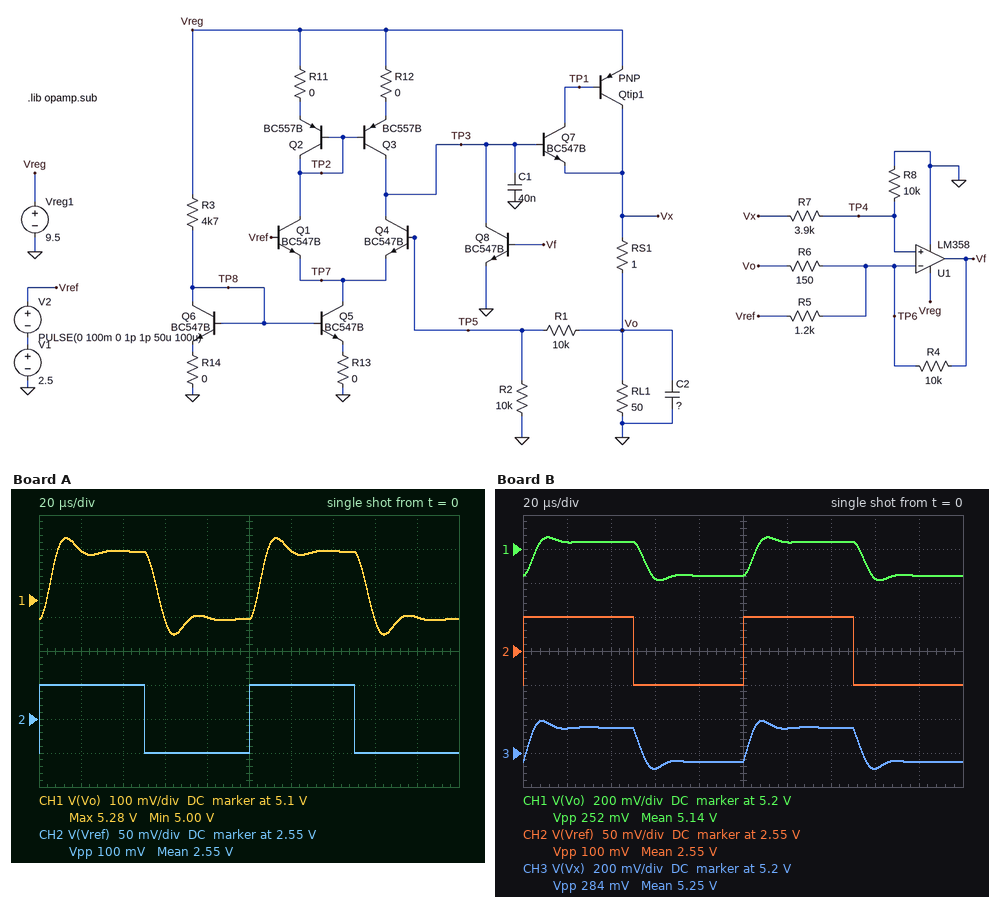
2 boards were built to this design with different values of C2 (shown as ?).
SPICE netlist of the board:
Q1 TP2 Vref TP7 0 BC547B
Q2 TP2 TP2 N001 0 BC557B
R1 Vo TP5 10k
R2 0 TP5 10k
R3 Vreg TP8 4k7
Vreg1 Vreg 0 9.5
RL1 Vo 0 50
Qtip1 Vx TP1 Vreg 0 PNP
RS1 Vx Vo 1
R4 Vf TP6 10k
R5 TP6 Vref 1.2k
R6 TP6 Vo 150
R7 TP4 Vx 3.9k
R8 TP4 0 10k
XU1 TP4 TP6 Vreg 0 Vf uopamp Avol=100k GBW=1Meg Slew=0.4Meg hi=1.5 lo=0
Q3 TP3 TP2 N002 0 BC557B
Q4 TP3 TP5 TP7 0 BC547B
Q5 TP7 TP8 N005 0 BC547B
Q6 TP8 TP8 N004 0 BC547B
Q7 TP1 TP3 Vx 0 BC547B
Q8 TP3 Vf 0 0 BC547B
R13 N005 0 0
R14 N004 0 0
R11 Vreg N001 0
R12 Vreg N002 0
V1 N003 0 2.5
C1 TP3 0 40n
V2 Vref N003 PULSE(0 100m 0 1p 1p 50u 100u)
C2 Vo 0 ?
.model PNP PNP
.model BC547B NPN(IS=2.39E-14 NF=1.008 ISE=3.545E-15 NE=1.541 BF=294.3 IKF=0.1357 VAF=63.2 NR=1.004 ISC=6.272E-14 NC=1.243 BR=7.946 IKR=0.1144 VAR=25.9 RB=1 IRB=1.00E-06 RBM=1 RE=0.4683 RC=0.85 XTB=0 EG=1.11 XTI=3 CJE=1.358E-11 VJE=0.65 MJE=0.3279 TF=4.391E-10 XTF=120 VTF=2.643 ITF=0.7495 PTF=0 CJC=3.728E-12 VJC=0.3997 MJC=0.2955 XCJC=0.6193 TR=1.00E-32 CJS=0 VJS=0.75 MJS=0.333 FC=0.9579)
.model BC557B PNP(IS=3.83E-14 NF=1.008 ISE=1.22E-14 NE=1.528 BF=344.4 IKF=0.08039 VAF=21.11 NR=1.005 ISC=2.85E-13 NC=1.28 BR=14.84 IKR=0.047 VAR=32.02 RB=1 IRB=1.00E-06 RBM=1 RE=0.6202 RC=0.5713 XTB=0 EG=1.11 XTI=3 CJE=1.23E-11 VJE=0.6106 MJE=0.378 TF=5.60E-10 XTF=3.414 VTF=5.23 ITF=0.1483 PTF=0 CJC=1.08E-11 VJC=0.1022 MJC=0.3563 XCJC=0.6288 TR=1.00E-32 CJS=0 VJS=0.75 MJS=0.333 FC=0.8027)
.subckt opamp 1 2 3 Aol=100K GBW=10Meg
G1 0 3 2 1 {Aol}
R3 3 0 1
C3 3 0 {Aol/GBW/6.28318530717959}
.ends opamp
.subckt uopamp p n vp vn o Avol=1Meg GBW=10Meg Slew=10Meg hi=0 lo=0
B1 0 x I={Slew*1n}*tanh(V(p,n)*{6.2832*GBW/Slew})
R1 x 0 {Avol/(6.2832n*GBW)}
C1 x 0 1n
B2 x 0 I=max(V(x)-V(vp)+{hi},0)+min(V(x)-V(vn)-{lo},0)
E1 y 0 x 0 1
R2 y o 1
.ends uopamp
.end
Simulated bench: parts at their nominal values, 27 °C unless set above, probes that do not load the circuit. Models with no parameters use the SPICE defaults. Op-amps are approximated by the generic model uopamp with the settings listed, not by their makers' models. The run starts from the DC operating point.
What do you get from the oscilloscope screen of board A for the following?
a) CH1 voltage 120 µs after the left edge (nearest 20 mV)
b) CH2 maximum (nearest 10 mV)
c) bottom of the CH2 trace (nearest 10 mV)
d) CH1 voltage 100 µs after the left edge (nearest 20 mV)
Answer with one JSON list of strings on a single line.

["5.24 V", "2.60 V", "2.50 V", "5.04 V"]
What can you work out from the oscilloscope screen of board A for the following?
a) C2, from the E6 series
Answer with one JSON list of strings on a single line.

["3.3 µF"]
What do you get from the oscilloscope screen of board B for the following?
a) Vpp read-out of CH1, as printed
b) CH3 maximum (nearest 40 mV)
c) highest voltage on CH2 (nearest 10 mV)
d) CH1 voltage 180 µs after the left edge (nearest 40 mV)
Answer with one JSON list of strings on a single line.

["252 mV", "5.40 V", "2.60 V", "5.04 V"]
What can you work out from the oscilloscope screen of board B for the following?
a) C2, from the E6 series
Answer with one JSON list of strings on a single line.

["2.2 µF"]
